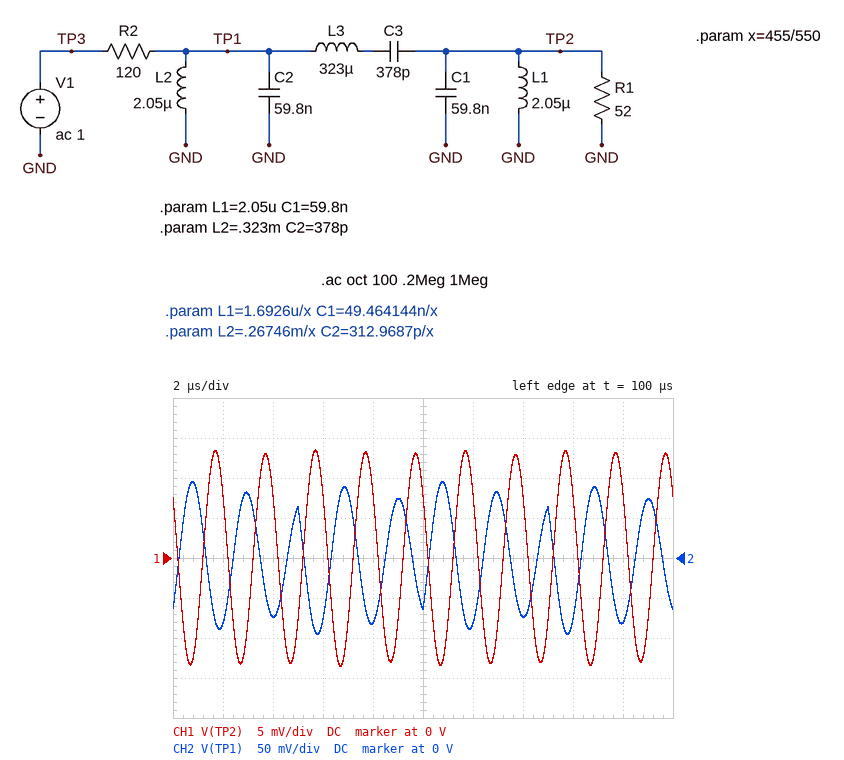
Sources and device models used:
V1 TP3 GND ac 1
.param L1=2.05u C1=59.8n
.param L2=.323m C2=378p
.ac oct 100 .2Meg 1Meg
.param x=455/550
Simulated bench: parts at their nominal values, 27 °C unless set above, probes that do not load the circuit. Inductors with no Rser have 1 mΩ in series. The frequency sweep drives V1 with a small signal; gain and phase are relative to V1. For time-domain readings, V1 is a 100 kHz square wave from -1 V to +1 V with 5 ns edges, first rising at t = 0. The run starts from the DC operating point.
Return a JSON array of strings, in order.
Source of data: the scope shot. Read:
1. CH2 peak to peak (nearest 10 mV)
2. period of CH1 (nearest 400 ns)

["190 mV", "2.0 µs"]
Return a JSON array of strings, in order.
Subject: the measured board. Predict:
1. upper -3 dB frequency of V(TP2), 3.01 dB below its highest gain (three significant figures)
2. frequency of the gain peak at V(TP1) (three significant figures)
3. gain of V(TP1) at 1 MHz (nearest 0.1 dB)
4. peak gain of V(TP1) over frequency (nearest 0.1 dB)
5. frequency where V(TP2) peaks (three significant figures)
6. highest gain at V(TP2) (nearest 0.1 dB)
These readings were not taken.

["483 kHz", "431 kHz", "-31.1 dB", "-4.6 dB", "437 kHz", "-9.7 dB"]
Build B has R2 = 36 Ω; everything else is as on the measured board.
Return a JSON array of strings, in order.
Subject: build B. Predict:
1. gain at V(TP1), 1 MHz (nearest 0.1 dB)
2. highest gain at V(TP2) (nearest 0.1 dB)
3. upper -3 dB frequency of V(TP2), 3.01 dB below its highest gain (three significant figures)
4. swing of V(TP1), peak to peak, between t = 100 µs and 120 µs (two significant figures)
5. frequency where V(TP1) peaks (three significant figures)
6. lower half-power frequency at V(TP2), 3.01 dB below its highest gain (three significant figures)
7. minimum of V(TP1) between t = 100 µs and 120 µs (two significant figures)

["-20.6 dB", "-4.6 dB", "480 kHz", "600 mV", "428 kHz", "432 kHz", "-300 mV"]
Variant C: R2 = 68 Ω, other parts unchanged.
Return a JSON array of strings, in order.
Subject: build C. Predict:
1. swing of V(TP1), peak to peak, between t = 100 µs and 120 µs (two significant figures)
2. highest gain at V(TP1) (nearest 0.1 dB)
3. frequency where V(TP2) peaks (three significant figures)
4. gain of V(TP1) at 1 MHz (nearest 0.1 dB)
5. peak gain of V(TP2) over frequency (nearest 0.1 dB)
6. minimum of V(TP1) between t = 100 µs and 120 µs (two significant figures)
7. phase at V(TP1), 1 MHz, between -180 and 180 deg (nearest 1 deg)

["340 mV", "-2.7 dB", "469 kHz", "-26.1 dB", "-7.2 dB", "-170 mV", "-87 deg"]
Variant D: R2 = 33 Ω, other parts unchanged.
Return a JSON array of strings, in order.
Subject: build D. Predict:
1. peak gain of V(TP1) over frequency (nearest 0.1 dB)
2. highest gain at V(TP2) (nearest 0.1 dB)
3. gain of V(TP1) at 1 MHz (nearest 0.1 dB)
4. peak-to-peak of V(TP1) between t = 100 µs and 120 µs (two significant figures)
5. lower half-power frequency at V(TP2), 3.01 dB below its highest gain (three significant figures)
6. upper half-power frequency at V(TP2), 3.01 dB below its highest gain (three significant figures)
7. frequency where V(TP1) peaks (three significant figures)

["-1.2 dB", "-4.3 dB", "-19.9 dB", "650 mV", "432 kHz", "479 kHz", "428 kHz"]
